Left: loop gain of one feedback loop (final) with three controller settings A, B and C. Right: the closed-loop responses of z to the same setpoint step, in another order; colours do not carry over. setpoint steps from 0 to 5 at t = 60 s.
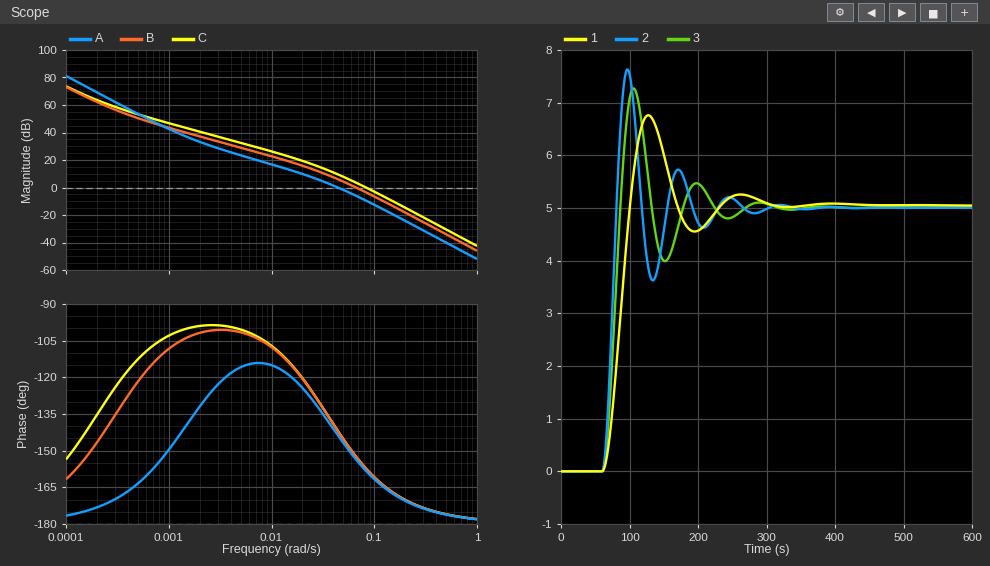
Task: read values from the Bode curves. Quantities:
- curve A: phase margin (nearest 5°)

35°
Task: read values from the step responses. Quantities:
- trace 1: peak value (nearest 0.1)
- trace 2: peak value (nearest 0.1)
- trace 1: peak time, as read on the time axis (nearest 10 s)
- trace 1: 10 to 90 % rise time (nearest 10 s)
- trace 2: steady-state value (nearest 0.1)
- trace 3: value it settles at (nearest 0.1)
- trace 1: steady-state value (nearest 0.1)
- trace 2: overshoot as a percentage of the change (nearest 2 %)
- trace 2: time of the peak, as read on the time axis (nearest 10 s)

6.8
7.6
130 s
30 s
5.0
5.0
5.0
52 %
100 s
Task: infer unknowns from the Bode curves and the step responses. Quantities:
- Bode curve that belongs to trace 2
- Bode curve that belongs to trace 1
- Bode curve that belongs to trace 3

C
A
B
